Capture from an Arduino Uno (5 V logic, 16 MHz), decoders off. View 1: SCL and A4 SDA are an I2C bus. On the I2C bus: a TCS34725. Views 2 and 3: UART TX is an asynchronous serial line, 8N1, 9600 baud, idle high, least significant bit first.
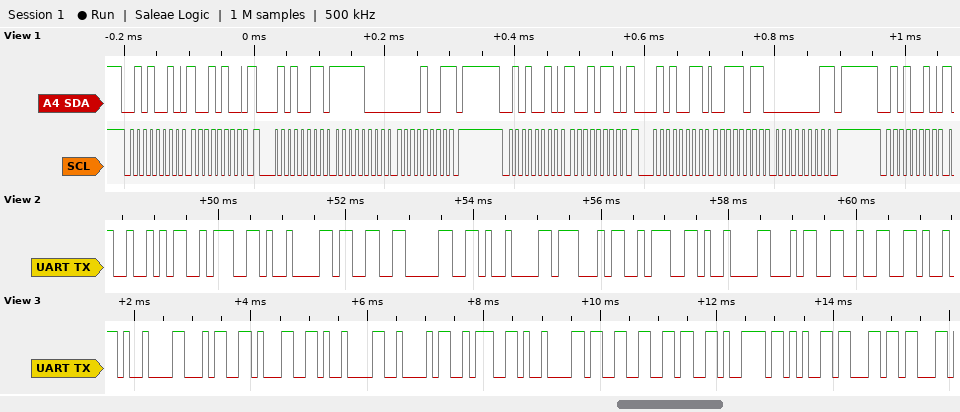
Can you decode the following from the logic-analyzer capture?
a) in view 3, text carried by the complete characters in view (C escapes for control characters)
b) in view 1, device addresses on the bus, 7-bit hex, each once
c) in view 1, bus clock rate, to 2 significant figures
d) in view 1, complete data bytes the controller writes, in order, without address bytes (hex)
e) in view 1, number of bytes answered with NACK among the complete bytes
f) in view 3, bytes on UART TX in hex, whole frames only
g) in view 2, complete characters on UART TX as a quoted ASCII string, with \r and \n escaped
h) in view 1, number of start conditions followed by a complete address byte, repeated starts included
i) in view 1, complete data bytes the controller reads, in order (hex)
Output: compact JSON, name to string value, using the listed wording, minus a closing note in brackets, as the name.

{"in view 3, text carried by the complete characters in view": "\"\\t41\\tB:\\t36yel\"", "in view 1, device addresses on the bus, 7-bit hex, each once": "0x29", "in view 1, bus clock rate, to 2 significant figures": "100 kHz", "in view 1, complete data bytes the controller writes, in order, without address bytes": "94 96", "in view 1, number of bytes answered with NACK among the complete bytes": "2", "in view 3, bytes on UART TX in hex, whole frames only": "09 34 31 09 42 3A 09 33 36 79 65 6C", "in view 2, complete characters on UART TX as a quoted ASCII string, with \\r and \\n escaped": "\"R:\\t30\\tG:\\t42\"", "in view 1, number of start conditions followed by a complete address byte, repeated starts included": "5", "in view 1, complete data bytes the controller reads, in order": "F8 09 3B 01"}
